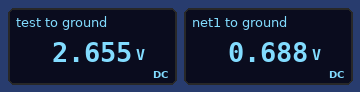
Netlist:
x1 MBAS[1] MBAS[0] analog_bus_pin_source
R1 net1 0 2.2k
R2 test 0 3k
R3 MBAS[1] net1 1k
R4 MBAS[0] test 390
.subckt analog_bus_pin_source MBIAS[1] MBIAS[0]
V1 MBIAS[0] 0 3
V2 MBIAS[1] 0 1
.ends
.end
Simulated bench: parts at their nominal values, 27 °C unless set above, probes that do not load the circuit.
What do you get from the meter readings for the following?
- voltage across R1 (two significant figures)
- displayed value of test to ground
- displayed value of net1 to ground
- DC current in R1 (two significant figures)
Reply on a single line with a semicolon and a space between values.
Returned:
690 mV; 2.655 V; 0.688 V; 310 µA
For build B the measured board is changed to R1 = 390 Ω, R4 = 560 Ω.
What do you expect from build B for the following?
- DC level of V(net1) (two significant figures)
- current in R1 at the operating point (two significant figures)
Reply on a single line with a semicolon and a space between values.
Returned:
280 mV; 720 µA
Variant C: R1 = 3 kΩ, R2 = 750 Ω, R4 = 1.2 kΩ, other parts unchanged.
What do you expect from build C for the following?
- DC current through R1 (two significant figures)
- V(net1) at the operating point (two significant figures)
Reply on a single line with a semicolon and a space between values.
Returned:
250 µA; 750 mV
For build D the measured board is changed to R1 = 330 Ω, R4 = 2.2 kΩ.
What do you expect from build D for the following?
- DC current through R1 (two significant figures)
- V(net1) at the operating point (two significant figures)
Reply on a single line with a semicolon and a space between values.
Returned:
750 µA; 250 mV
